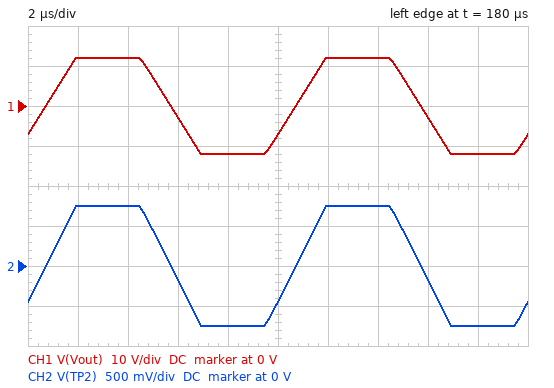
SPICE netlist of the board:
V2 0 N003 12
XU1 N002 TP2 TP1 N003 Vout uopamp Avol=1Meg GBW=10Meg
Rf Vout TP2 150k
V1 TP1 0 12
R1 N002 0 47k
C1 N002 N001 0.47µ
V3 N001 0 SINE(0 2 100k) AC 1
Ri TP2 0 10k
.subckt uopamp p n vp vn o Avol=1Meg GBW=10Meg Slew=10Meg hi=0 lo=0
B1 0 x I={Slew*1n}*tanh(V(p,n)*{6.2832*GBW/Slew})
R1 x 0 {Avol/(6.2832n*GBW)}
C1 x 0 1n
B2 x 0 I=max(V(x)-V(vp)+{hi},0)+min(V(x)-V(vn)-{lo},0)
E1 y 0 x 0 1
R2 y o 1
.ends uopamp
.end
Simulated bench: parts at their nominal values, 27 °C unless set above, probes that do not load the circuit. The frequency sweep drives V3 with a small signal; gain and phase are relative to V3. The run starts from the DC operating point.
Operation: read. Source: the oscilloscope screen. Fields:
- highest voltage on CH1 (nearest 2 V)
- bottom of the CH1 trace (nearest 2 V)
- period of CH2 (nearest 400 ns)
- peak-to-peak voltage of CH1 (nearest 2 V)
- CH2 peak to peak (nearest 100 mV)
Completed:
12 V
-12 V
10.0 µs
24 V
1.5 V
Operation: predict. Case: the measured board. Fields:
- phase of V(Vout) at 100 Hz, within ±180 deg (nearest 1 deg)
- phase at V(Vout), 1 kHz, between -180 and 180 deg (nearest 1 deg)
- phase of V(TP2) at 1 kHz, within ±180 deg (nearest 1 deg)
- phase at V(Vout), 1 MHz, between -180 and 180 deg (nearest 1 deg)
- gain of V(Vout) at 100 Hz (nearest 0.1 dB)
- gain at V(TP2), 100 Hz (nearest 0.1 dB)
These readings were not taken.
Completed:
4 deg
0 deg
0 deg
-58 deg
24.1 dB
0 dB
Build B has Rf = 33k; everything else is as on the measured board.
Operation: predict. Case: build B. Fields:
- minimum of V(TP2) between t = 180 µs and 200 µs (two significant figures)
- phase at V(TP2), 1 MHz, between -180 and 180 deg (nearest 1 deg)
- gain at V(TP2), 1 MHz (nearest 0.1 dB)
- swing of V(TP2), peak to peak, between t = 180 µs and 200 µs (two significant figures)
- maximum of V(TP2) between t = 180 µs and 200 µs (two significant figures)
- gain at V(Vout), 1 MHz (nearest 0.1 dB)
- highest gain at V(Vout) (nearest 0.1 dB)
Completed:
-2.0 V
-23 deg
-0.7 dB
4.0 V
2.0 V
11.9 dB
12.7 dB
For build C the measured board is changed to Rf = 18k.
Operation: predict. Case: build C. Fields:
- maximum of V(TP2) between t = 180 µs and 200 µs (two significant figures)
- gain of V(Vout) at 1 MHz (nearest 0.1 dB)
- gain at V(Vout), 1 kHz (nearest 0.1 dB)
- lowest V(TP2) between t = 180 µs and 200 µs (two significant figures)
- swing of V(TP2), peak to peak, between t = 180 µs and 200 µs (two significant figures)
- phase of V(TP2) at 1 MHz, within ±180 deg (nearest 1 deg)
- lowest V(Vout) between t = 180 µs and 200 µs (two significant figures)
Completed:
2.0 V
8.6 dB
8.9 dB
-2.0 V
4.0 V
-16 deg
-5.6 V
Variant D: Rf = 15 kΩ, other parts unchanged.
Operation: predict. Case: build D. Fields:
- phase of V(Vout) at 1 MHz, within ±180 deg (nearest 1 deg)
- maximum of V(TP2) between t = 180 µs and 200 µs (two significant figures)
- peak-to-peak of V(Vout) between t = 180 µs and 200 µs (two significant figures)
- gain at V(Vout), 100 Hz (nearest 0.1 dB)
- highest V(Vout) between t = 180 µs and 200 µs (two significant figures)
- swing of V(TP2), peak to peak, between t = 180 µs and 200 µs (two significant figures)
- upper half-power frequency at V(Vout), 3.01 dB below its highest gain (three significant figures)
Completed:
-14 deg
2.0 V
10 V
7.9 dB
5.0 V
4.0 V
4.00 MHz
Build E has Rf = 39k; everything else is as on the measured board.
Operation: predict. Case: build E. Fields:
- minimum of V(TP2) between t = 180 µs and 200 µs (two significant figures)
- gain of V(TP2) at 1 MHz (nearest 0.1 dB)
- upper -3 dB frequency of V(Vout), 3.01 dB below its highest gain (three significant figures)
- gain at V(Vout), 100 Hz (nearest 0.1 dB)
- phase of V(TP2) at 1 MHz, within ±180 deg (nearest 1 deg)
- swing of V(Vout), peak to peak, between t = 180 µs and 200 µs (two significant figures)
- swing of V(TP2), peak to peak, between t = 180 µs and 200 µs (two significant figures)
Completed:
-2.0 V
-0.9 dB
2.04 MHz
13.8 dB
-26 deg
20 V
4.0 V
